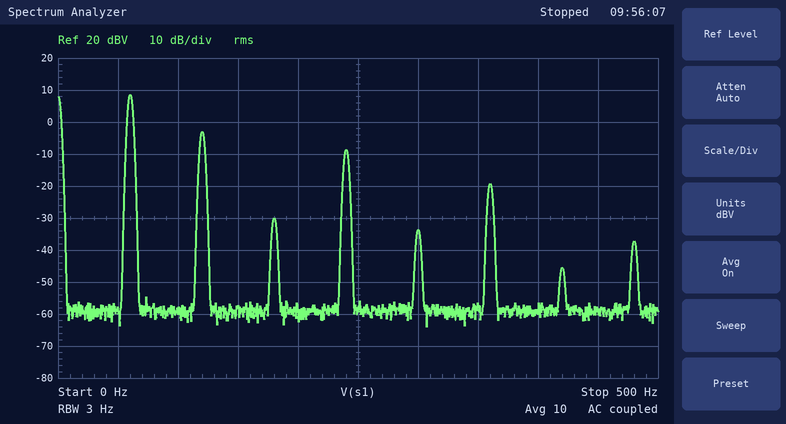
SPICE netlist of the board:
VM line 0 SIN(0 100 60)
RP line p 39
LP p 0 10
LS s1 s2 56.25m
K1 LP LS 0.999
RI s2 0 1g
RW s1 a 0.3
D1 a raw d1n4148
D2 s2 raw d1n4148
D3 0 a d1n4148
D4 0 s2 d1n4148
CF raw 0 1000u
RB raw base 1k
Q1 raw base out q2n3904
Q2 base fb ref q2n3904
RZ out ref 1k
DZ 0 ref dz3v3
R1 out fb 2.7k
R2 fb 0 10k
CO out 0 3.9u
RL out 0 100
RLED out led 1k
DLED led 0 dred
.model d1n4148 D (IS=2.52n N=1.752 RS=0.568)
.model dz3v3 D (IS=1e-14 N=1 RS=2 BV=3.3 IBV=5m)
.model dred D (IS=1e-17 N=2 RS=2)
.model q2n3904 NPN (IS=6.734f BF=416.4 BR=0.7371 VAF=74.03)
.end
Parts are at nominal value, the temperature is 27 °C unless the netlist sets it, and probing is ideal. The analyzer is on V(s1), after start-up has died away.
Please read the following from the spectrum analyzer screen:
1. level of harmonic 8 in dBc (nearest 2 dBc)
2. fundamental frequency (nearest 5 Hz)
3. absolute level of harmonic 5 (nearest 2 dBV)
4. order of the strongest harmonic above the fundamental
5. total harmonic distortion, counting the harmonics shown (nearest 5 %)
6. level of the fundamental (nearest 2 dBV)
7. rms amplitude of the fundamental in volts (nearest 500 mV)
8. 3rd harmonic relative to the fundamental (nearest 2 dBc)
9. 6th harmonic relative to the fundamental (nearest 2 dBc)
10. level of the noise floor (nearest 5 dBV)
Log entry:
-46 dBc
60 Hz
-34 dBV
2
30 %
8 dBV
2.5 V
-38 dBc
-28 dBc
-60 dBV
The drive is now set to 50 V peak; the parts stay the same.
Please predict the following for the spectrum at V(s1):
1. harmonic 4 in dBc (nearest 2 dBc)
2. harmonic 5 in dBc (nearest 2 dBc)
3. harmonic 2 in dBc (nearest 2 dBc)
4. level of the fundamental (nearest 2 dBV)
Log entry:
-20 dBc
-38 dBc
-16 dBc
2 dBV
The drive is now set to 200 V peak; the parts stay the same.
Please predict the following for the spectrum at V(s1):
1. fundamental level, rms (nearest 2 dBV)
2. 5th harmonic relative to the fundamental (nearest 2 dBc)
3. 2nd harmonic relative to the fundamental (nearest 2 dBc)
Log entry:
14 dBV
-54 dBc
-10 dBc
